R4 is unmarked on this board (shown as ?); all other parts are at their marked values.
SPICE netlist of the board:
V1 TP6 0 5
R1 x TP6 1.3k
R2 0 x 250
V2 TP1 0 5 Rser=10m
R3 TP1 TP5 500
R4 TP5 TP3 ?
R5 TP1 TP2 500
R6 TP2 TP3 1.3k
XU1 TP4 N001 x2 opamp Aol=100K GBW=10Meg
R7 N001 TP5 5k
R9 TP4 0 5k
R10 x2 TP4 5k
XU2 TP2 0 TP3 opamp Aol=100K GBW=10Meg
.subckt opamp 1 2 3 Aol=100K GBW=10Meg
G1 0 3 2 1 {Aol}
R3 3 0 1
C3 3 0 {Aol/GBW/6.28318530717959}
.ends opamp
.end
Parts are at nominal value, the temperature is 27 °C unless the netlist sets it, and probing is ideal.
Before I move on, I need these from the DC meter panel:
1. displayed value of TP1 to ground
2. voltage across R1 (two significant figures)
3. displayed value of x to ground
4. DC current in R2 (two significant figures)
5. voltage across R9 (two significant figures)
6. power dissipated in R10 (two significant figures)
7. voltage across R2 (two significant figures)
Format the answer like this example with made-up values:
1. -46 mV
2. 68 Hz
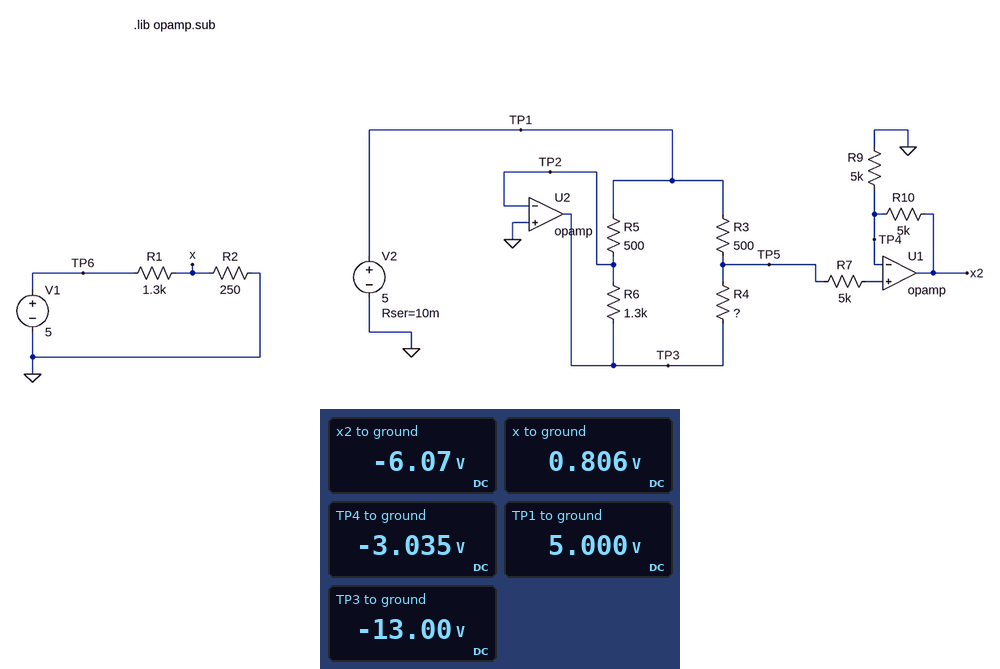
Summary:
1. 5.000 V
2. 4.2 V
3. 0.806 V
4. 3.2 mA
5. 3.0 V
6. 1.8 mW
7. 810 mV
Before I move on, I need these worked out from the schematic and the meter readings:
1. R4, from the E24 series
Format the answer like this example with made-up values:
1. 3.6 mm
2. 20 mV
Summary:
1. 620 Ω
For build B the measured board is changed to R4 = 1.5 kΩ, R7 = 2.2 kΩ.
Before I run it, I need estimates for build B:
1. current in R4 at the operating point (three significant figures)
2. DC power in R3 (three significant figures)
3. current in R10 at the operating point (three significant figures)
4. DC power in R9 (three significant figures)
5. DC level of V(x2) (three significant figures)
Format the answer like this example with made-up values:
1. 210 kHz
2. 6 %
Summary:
1. 9.00 mA
2. 40.5 mW
3. 100 µA
4. 50.0 µW
5. 1.00 V
